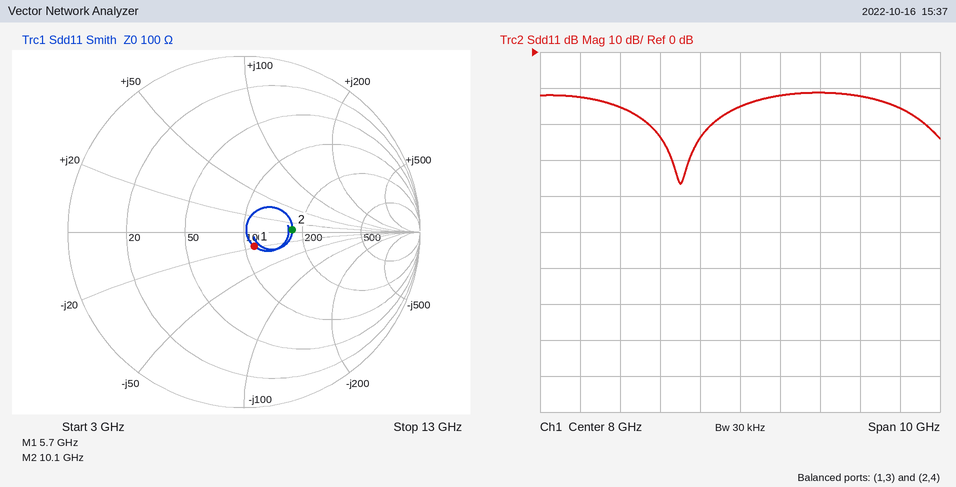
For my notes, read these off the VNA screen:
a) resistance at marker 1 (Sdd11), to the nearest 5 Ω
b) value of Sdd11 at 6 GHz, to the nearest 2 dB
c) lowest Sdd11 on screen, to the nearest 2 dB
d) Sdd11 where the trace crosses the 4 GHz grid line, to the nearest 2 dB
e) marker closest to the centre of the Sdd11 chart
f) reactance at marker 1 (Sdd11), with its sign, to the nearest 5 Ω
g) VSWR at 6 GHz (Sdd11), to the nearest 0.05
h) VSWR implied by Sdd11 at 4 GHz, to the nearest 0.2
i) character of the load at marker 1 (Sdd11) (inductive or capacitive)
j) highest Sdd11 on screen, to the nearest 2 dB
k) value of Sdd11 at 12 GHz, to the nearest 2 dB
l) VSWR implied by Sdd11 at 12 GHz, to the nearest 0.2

110 Ω
-24 dB
-36 dB
-12 dB
marker 1
-20 Ω
1.15
1.6
capacitive
-12 dB
-16 dB
1.4
